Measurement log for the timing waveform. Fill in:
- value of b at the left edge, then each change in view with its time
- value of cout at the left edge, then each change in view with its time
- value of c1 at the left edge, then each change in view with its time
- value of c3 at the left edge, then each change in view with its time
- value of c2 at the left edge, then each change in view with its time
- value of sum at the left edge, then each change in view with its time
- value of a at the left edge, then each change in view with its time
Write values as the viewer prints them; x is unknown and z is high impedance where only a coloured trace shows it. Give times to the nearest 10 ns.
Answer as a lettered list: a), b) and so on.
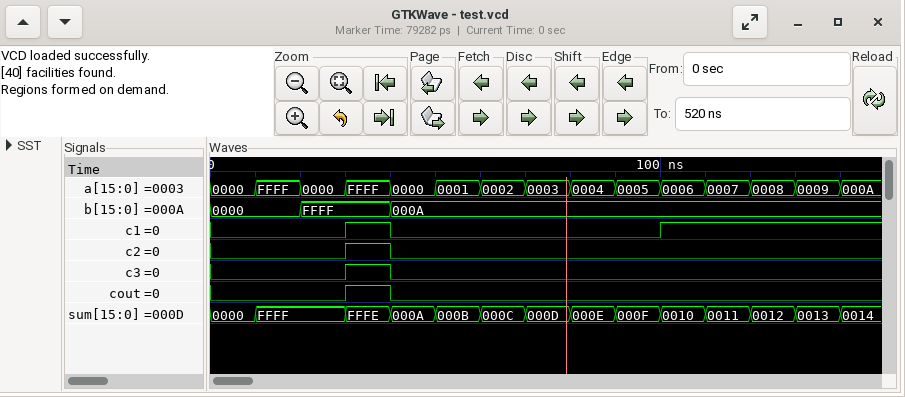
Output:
a) 0000, FFFF at 20 ns, 000A at 40 ns
b) 0, 1 at 30 ns, 0 at 40 ns
c) 0, 1 at 30 ns, 0 at 40 ns, 1 at 100 ns
d) 0, 1 at 30 ns, 0 at 40 ns
e) 0, 1 at 30 ns, 0 at 40 ns
f) 0000, FFFF at 10 ns, FFFE at 30 ns, 000A at 40 ns, 000B at 50 ns, 000C at 60 ns, 000D at 70 ns, 000E at 80 ns, 000F at 90 ns, 0010 at 100 ns, 0011 at 110 ns, 0012 at 120 ns, 0013 at 130 ns, 0014 at 140 ns
g) 0000, FFFF at 10 ns, 0000 at 20 ns, FFFF at 30 ns, 0000 at 40 ns, 0001 at 50 ns, 0002 at 60 ns, 0003 at 70 ns, 0004 at 80 ns, 0005 at 90 ns, 0006 at 100 ns, 0007 at 110 ns, 0008 at 120 ns, 0009 at 130 ns, 000A at 140 ns
